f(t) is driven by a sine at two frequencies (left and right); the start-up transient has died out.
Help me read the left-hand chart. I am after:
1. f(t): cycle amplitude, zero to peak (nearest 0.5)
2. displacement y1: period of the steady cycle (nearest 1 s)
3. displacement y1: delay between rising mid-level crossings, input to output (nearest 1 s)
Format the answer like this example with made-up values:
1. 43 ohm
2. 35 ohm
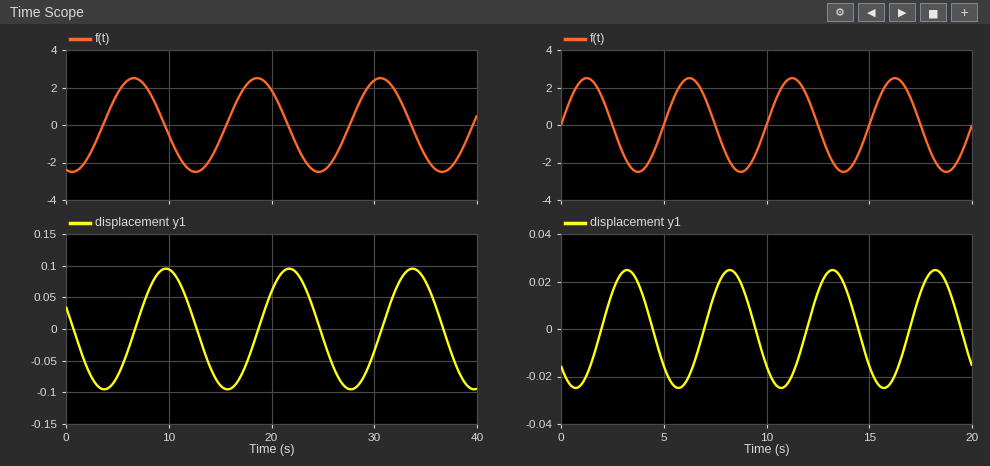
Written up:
1. 2.5
2. 12 s
3. 3 s
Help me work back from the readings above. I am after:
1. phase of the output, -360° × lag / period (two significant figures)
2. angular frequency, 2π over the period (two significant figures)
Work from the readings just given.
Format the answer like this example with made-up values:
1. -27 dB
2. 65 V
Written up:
1. -90°
2. 0.52 rad/s
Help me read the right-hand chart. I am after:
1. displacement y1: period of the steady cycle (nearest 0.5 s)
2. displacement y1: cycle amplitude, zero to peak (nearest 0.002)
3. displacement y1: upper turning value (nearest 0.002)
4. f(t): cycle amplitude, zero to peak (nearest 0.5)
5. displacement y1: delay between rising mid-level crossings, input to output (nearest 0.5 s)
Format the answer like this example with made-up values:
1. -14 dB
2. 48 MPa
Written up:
1. 5.0 s
2. 0.024
3. 0.024
4. 2.5
5. 2.0 s
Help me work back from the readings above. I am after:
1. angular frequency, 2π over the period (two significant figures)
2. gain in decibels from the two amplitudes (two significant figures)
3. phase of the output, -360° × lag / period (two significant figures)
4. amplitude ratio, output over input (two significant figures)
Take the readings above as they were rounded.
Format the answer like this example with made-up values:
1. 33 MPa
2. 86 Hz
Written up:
1. 1.3 rad/s
2. -40 dB
3. -140°
4. 0.0096
